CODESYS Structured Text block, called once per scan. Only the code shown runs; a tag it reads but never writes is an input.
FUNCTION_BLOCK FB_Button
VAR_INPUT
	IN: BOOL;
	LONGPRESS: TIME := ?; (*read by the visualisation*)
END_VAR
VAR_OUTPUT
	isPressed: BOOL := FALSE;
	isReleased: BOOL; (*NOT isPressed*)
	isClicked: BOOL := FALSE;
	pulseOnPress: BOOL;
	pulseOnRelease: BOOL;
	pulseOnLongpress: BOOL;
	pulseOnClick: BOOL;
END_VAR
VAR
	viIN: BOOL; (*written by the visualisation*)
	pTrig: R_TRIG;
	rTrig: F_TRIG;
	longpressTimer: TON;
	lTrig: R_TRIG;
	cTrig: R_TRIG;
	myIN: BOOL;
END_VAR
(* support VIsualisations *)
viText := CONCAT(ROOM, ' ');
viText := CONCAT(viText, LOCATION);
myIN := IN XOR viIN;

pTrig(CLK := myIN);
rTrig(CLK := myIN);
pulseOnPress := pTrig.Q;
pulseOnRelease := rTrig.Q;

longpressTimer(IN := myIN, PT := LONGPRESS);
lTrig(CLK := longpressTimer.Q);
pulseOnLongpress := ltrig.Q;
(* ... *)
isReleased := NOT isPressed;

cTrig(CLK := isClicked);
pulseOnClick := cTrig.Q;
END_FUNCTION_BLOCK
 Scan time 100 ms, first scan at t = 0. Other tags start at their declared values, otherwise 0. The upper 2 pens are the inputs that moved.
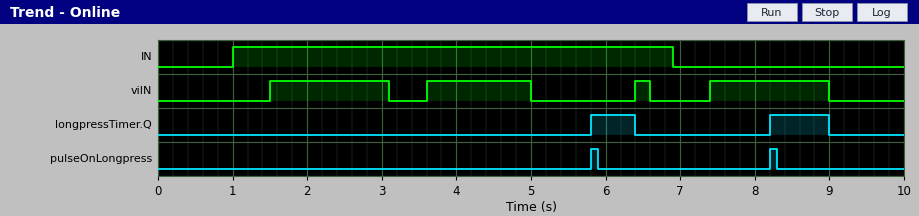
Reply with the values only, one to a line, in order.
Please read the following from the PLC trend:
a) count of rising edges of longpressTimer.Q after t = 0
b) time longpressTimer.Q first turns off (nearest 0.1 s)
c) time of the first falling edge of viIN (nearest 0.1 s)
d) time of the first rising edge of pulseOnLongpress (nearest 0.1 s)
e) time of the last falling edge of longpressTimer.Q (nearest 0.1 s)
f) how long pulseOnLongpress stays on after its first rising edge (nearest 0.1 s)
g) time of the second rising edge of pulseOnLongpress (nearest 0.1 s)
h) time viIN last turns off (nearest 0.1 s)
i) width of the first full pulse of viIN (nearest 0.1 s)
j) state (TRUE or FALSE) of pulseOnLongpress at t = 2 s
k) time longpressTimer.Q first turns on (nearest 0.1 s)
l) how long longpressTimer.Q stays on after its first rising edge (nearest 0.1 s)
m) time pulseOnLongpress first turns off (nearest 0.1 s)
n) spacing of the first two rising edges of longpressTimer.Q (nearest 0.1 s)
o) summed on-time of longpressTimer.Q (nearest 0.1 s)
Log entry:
2
6.4 s
3.1 s
5.8 s
9.0 s
0.1 s
8.2 s
9.0 s
1.6 s
FALSE
5.8 s
0.6 s
5.9 s
2.4 s
1.4 s
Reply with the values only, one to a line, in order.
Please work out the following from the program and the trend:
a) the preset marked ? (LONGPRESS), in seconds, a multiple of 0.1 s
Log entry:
0.8 s
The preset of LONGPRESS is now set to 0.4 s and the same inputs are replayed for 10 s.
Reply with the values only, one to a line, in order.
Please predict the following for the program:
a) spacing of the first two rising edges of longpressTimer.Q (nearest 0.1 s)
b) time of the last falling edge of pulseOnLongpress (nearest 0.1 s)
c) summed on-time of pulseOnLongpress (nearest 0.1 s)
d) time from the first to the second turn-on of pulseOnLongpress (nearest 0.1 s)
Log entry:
2.1 s
7.9 s
0.4 s
2.1 s
